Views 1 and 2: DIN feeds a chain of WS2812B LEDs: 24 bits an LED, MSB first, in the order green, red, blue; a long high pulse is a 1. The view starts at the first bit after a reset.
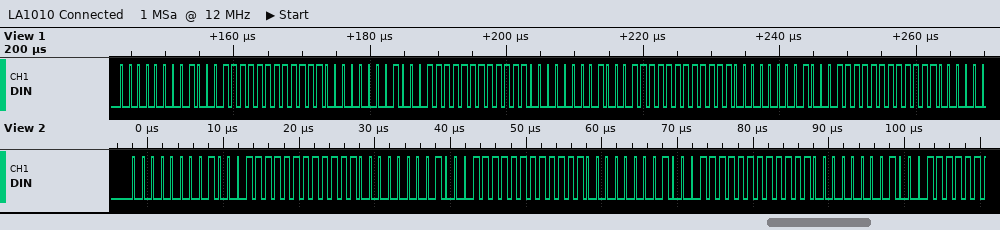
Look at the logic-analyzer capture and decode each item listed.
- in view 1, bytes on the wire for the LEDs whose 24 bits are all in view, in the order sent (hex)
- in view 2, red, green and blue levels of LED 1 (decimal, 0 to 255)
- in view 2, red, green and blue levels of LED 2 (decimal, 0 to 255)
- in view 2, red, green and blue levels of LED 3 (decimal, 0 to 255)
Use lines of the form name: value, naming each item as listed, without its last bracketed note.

in view 1, bytes on the wire for the LEDs whose 24 bits are all in view, in the order sent: 00 8F FF 00 8F FF 00 8F FF 00 8F FF
in view 2, red, green and blue levels of LED 1: 143, 0, 255
in view 2, red, green and blue levels of LED 2: 143, 0, 255
in view 2, red, green and blue levels of LED 3: 143, 0, 255
